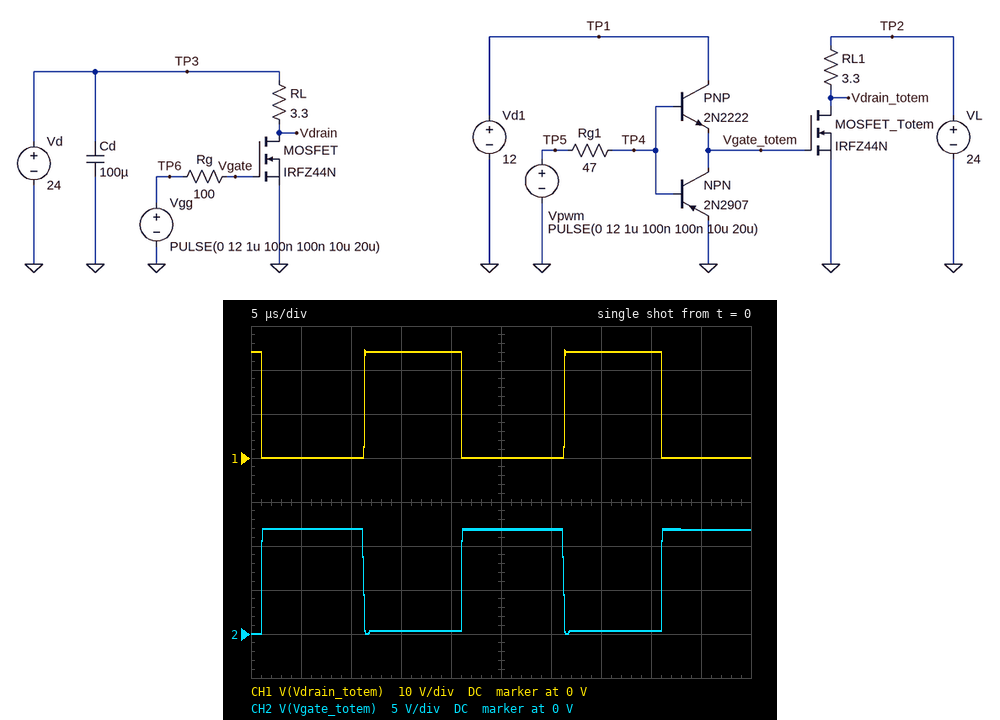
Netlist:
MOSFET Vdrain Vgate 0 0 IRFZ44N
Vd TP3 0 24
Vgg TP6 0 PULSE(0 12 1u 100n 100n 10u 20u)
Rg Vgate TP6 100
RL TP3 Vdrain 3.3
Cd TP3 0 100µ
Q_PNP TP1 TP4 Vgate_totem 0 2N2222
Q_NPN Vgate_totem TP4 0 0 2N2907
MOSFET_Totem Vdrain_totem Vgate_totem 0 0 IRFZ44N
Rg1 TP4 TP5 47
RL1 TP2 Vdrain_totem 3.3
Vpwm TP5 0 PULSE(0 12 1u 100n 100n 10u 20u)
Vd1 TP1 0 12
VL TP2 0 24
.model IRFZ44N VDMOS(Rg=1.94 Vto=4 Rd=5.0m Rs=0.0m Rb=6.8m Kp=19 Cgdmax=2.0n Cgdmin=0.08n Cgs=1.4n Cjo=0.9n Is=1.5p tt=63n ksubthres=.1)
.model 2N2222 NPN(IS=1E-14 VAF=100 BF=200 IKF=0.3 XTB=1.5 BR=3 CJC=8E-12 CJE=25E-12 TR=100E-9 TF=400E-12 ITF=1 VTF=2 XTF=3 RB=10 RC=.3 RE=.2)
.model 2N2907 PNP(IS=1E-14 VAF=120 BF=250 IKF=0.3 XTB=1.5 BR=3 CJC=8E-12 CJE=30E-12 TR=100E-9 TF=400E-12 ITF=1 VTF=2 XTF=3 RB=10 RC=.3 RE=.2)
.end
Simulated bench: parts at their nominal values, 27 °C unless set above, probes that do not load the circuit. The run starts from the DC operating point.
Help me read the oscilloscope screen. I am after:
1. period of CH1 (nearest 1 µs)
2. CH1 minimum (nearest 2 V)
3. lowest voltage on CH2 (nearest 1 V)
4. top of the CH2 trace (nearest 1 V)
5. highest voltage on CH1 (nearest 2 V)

20 µs
0 V
0 V
12 V
24 V
